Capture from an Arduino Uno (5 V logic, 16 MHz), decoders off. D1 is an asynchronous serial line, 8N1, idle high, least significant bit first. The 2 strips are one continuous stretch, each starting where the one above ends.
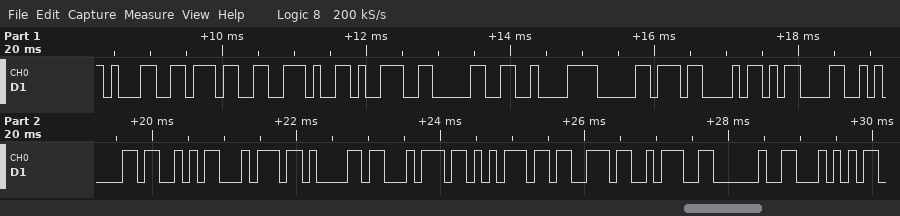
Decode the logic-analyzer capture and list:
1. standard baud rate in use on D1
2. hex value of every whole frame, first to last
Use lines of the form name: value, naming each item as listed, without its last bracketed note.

standard baud rate in use on D1: 9600 baud
hex value of every whole frame, first to last: 0x31 0x37 0x2E 0x39 0x30 0xC2 0xB0 0x43 0x0D 0x0A 0x53 0x74 0x61 0x74 0x75 0x73 0x3A 0x20 0x54
